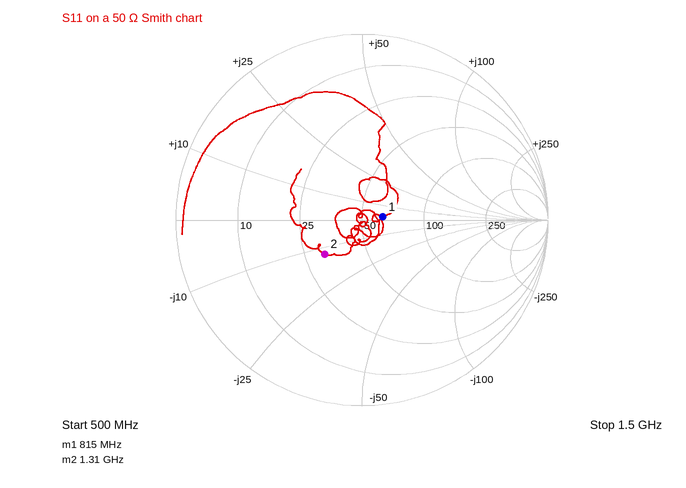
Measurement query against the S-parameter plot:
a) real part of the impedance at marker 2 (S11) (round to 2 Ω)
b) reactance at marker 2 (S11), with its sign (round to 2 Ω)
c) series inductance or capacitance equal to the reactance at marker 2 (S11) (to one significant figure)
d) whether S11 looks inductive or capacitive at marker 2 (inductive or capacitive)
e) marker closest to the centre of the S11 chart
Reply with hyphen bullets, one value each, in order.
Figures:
- 32 Ω
- -12 Ω
- 10 pF
- capacitive
- marker 1
